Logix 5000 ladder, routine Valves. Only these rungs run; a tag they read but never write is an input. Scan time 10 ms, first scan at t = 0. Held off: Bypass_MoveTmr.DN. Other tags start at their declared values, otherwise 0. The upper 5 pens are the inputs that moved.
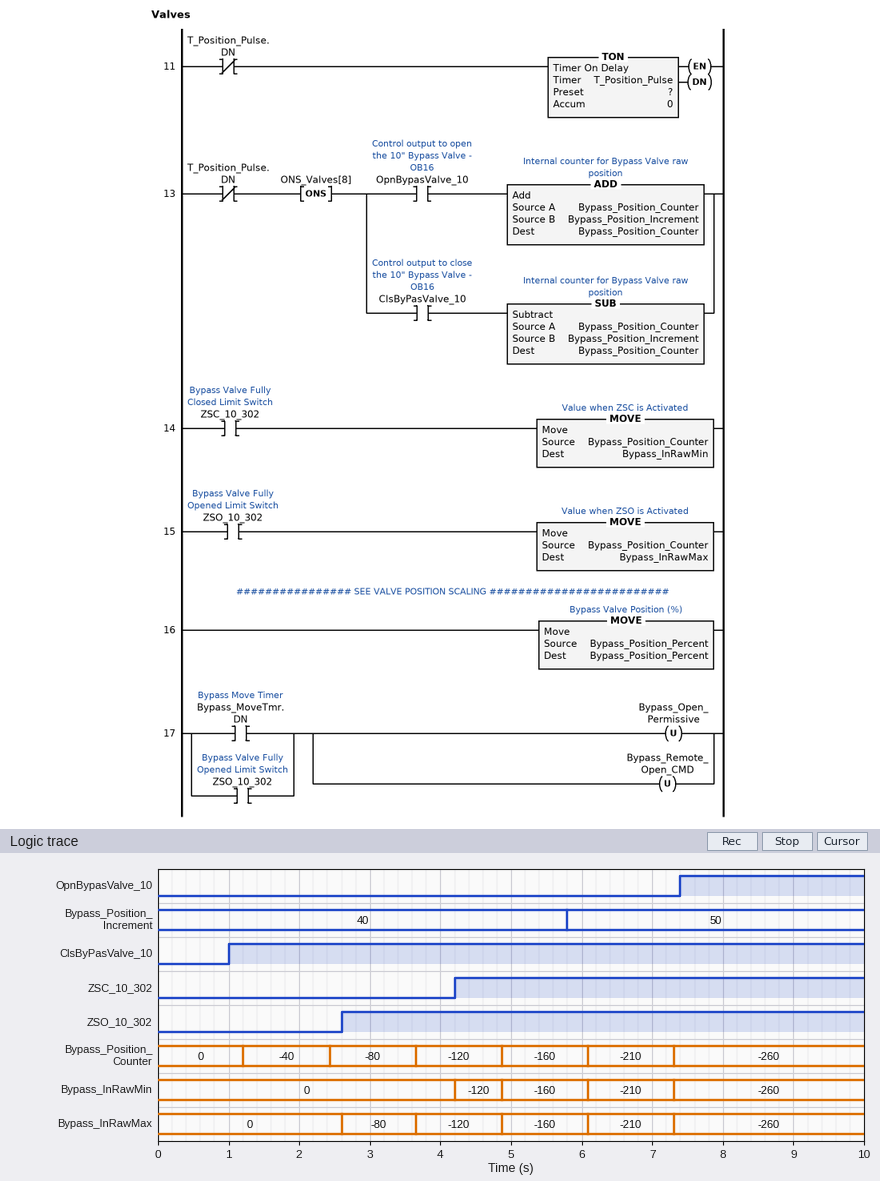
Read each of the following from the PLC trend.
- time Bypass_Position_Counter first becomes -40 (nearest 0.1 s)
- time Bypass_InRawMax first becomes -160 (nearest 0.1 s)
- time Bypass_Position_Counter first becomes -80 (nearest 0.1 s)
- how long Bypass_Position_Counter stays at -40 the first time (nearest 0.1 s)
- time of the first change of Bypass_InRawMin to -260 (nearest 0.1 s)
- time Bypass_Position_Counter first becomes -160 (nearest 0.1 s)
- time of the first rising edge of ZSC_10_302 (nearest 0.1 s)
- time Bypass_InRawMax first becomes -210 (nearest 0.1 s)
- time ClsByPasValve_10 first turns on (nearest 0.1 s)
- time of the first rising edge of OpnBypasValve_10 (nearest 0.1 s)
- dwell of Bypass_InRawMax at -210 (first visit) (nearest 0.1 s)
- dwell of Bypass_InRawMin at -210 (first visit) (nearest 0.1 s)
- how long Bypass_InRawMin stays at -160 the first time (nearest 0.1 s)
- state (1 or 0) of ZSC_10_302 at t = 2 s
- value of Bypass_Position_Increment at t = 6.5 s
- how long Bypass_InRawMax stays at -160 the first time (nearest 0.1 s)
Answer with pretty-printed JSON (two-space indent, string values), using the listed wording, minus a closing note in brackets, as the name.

{
  "time Bypass_Position_Counter first becomes -40": "1.2 s",
  "time Bypass_InRawMax first becomes -160": "4.9 s",
  "time Bypass_Position_Counter first becomes -80": "2.4 s",
  "how long Bypass_Position_Counter stays at -40 the first time": "1.2 s",
  "time of the first change of Bypass_InRawMin to -260": "7.3 s",
  "time Bypass_Position_Counter first becomes -160": "4.9 s",
  "time of the first rising edge of ZSC_10_302": "4.2 s",
  "time Bypass_InRawMax first becomes -210": "6.1 s",
  "time ClsByPasValve_10 first turns on": "1.0 s",
  "time of the first rising edge of OpnBypasValve_10": "7.4 s",
  "dwell of Bypass_InRawMax at -210 (first visit)": "1.2 s",
  "dwell of Bypass_InRawMin at -210 (first visit)": "1.2 s",
  "how long Bypass_InRawMin stays at -160 the first time": "1.2 s",
  "state (1 or 0) of ZSC_10_302 at t = 2 s": "0",
  "value of Bypass_Position_Increment at t = 6.5 s": "50",
  "how long Bypass_InRawMax stays at -160 the first time": "1.2 s"
}
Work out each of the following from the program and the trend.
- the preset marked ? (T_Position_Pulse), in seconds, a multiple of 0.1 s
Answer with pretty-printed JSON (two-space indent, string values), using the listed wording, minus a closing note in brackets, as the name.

{
  "the preset marked ? (T_Position_Pulse), in seconds, a multiple of 0.1 s": "1.2 s"
}
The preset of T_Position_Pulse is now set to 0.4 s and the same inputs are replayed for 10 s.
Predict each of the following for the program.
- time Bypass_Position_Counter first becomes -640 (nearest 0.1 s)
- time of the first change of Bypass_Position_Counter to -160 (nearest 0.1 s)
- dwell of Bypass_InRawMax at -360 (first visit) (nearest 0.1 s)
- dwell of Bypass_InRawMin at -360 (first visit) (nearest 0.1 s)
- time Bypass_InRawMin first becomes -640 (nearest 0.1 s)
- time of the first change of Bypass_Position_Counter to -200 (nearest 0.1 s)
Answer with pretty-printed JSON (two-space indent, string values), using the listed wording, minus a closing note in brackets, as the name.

{
  "time Bypass_Position_Counter first becomes -640": "7.1 s",
  "time of the first change of Bypass_Position_Counter to -160": "2.5 s",
  "dwell of Bypass_InRawMax at -360 (first visit)": "0.4 s",
  "dwell of Bypass_InRawMin at -360 (first visit)": "0.4 s",
  "time Bypass_InRawMin first becomes -640": "7.1 s",
  "time of the first change of Bypass_Position_Counter to -200": "2.9 s"
}
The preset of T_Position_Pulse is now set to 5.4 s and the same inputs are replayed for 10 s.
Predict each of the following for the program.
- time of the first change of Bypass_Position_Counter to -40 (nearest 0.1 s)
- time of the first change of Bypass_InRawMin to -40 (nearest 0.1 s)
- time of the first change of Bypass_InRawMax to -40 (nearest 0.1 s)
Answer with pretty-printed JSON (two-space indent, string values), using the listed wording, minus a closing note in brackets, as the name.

{
  "time of the first change of Bypass_Position_Counter to -40": "5.4 s",
  "time of the first change of Bypass_InRawMin to -40": "5.4 s",
  "time of the first change of Bypass_InRawMax to -40": "5.4 s"
}
